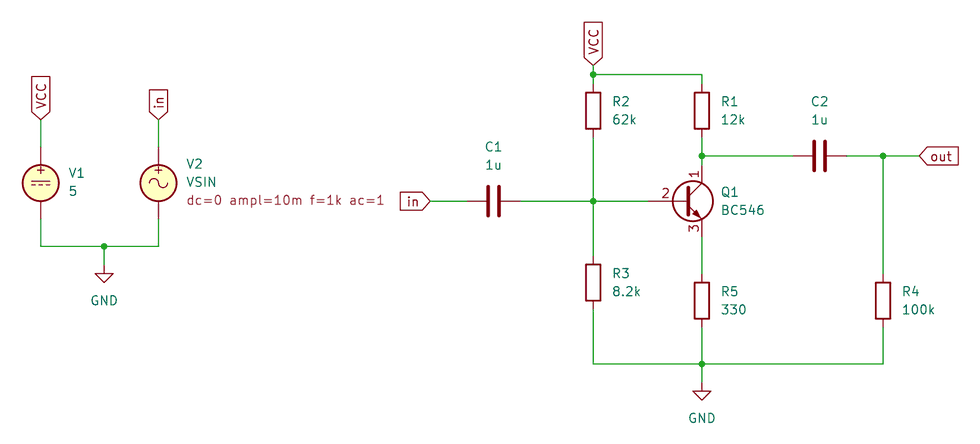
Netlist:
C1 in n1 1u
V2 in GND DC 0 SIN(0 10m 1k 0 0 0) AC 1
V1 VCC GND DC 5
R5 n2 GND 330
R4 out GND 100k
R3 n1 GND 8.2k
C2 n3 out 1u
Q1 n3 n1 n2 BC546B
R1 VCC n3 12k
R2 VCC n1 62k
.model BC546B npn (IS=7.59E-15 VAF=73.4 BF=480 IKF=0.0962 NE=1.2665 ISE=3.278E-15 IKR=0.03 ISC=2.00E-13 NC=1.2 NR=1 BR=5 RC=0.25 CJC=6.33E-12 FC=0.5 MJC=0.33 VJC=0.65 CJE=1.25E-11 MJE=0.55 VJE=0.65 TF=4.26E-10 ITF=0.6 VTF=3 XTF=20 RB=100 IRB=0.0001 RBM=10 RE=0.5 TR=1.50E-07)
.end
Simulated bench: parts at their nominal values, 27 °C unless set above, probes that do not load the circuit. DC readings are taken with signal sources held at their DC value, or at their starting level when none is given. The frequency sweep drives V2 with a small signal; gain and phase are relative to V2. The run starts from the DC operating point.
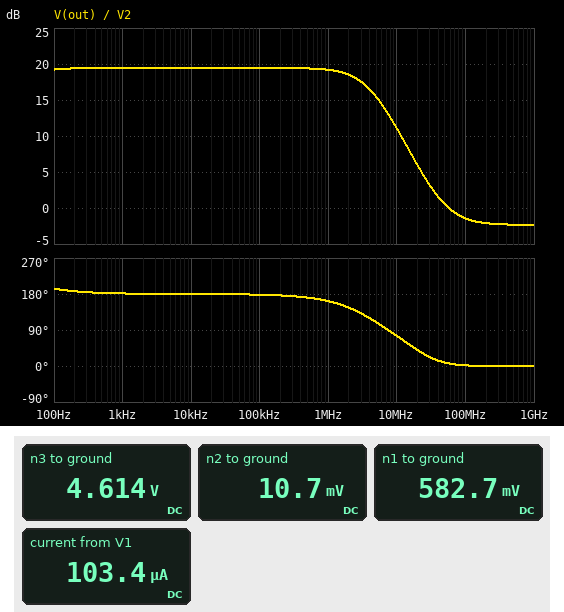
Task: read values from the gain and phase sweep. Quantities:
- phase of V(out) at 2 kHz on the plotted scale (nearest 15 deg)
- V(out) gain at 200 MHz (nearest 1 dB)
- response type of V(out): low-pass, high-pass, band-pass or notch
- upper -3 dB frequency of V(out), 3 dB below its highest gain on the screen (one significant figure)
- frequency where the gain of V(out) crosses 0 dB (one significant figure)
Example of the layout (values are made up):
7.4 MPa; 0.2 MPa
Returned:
180 deg; -2 dB; low-pass; 4 MHz; 60 MHz
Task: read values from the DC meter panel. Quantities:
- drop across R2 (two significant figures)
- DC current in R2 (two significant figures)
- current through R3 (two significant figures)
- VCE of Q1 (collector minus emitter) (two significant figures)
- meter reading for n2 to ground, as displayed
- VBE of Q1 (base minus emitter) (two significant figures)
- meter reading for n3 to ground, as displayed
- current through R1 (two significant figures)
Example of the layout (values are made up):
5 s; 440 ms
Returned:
4.4 V; 71 µA; 71 µA; 4.6 V; 10.7 mV; 570 mV; 4.614 V; 32 µA
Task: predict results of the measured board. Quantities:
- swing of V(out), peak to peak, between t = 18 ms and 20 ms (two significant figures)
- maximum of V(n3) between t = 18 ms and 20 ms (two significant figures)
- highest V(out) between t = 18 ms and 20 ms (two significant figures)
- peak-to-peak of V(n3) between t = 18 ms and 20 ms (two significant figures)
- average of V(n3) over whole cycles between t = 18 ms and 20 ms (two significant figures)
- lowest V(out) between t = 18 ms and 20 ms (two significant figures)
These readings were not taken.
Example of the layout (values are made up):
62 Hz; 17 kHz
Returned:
190 mV; 4.7 V; 86 mV; 190 mV; 4.6 V; -100 mV
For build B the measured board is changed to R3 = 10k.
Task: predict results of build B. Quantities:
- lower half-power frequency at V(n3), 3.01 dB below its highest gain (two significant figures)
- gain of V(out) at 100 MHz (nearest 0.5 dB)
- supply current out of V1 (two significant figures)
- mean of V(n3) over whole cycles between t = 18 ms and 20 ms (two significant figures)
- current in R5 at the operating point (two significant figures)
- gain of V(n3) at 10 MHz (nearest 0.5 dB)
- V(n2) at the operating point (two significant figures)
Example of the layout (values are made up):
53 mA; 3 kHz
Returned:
20 Hz; 0.5 dB; 270 µA; 2.6 V; 200 µA; 16.5 dB; 66 mV
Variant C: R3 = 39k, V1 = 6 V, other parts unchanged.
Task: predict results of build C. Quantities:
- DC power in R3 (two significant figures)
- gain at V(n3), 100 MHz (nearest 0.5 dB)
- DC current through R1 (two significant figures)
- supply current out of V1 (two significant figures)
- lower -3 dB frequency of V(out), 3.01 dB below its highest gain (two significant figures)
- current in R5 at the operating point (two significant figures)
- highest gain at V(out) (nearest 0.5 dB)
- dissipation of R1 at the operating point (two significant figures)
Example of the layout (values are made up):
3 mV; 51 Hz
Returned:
18 µW; -1.5 dB; 480 µA; 560 µA; 800 kHz; 540 µA; -1.5 dB; 2.8 mW
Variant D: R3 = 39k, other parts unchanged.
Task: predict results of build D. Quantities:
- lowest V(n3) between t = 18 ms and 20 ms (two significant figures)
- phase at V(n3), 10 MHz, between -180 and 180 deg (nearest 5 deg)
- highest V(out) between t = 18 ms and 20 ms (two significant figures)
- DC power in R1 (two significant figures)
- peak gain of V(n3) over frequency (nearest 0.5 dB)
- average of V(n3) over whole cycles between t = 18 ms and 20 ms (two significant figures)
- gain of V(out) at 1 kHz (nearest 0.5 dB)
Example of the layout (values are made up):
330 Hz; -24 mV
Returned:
200 mV; 5 deg; 6.3 mV; 1.9 mW; -1.5 dB; 210 mV; -9.5 dB
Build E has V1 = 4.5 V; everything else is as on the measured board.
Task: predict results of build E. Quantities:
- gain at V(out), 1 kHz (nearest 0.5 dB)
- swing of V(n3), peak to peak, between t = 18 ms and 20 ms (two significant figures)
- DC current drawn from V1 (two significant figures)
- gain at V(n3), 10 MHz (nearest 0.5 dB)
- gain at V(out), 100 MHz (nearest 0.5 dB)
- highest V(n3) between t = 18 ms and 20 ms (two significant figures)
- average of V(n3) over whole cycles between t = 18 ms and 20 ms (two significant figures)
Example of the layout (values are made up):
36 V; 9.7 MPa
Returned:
5.5 dB; 39 mV; 69 µA; 2.0 dB; -2.0 dB; 4.5 V; 4.4 V
